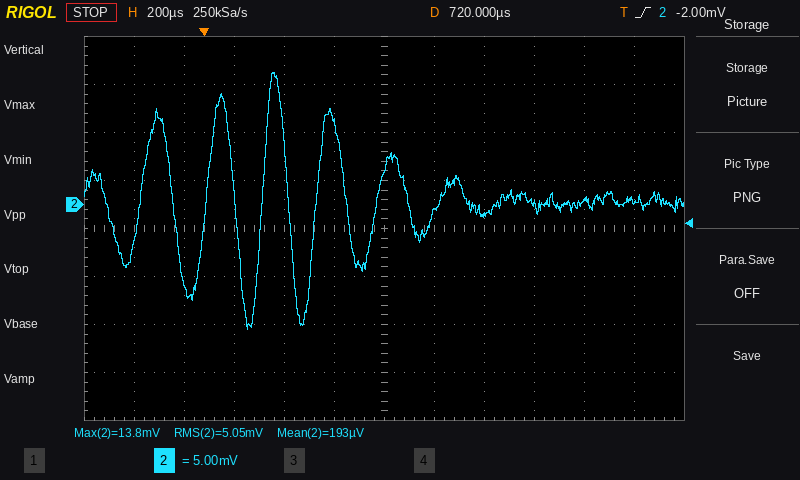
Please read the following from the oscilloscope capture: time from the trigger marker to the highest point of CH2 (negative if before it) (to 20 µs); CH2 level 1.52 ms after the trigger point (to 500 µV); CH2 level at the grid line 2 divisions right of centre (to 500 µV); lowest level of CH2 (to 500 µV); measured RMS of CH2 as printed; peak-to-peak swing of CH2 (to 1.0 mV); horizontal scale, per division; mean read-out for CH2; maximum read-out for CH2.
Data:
+280 µs
500 µV
-1.0 mV
-13.0 mV
5.05 mV
27.0 mV
200 µs
193 µV
13.8 mV
